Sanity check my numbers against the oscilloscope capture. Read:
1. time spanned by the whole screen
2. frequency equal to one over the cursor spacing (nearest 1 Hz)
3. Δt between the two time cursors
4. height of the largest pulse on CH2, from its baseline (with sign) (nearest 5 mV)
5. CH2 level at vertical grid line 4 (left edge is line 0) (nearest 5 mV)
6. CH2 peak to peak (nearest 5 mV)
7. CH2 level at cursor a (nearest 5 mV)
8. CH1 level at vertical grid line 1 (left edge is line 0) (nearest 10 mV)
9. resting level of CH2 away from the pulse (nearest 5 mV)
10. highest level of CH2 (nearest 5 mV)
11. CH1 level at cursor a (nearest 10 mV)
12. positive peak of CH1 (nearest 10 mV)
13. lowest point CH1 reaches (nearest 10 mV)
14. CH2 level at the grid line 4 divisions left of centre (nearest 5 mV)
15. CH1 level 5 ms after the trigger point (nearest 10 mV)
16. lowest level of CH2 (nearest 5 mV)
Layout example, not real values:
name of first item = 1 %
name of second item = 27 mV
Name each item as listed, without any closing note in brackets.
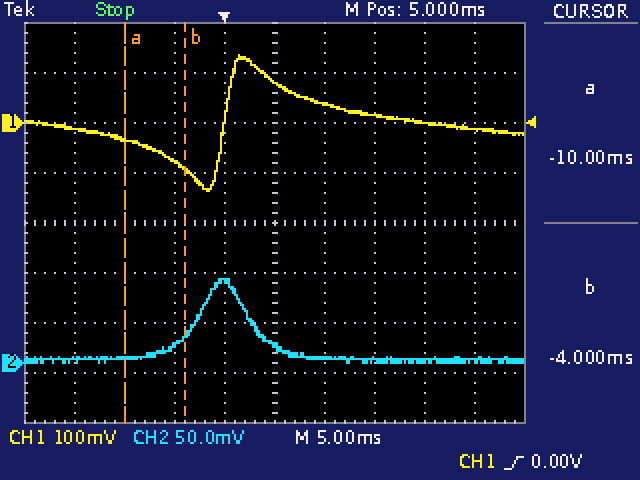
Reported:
time spanned by the whole screen = 50 ms
frequency equal to one over the cursor spacing = 167 Hz
Δt between the two time cursors = 6.0 ms
height of the largest pulse on CH2, from its baseline (with sign) = +80 mV
CH2 level at vertical grid line 4 (left edge is line 0) = 80 mV
CH2 peak to peak = 85 mV
CH2 level at cursor a = 5 mV
CH1 level at vertical grid line 1 (left edge is line 0) = -10 mV
resting level of CH2 away from the pulse = 5 mV
highest level of CH2 = 85 mV
CH1 level at cursor a = -30 mV
positive peak of CH1 = 140 mV
lowest point CH1 reaches = -140 mV
CH2 level at the grid line 4 divisions left of centre = 5 mV
CH1 level 5 ms after the trigger point = 80 mV
lowest level of CH2 = 0 mV
